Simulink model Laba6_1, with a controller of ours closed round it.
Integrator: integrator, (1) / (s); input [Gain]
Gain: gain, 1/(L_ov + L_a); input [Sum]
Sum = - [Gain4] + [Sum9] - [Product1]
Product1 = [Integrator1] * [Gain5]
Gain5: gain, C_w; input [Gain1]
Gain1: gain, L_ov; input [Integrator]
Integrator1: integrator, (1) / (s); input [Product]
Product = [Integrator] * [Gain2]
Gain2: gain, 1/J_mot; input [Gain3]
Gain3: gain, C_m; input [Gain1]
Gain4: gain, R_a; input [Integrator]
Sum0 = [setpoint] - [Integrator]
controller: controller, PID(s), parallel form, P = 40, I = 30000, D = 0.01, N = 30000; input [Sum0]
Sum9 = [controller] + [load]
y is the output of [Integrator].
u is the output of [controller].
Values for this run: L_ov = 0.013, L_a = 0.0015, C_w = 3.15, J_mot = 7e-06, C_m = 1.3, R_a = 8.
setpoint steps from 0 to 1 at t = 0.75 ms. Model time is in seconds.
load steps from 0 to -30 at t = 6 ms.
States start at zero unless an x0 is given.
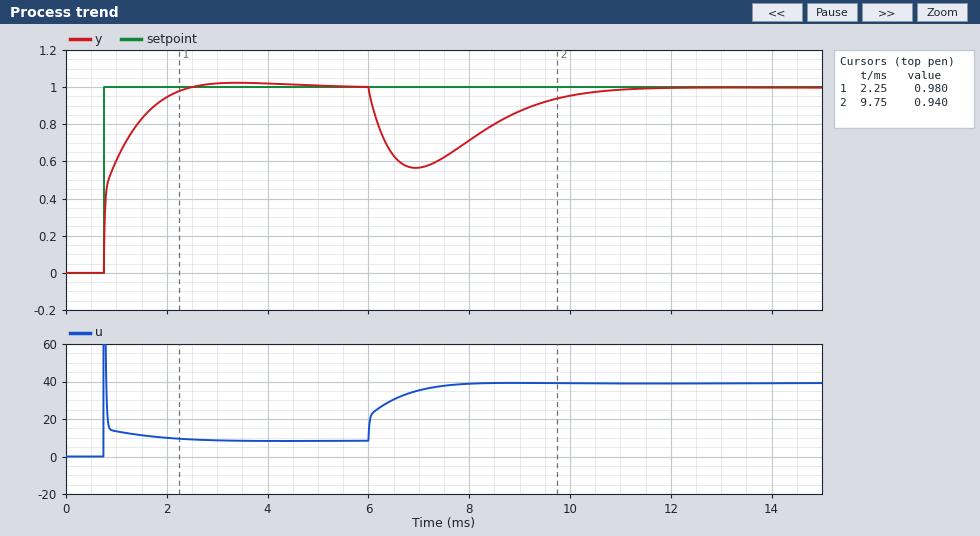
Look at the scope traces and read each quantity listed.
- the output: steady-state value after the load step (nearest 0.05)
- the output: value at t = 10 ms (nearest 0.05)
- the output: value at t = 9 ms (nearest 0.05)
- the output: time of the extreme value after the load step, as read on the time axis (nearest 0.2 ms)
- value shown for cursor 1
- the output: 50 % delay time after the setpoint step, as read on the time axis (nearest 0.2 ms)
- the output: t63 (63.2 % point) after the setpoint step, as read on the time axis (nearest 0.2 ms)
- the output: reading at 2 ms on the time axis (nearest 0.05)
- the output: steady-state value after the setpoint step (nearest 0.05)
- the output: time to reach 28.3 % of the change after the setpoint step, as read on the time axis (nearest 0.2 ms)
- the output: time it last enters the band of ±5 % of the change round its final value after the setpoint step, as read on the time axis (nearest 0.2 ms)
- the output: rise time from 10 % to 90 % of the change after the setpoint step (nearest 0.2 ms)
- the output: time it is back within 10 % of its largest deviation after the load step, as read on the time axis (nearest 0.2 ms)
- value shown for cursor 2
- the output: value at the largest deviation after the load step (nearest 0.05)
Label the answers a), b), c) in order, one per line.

a) 1.00
b) 0.95
c) 0.85
d) 7.0 ms
e) 0.980
f) 0.8 ms
g) 1.0 ms
h) 0.95
i) 1.00
j) 0.8 ms
k) 2.0 ms
l) 1.0 ms
m) 10.0 ms
n) 0.940
o) 0.55
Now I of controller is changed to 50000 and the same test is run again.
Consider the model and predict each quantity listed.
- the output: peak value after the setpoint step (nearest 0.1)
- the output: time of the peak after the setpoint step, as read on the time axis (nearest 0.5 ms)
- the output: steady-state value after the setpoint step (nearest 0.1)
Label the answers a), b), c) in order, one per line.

a) 1.1
b) 2.5 ms
c) 1.0
